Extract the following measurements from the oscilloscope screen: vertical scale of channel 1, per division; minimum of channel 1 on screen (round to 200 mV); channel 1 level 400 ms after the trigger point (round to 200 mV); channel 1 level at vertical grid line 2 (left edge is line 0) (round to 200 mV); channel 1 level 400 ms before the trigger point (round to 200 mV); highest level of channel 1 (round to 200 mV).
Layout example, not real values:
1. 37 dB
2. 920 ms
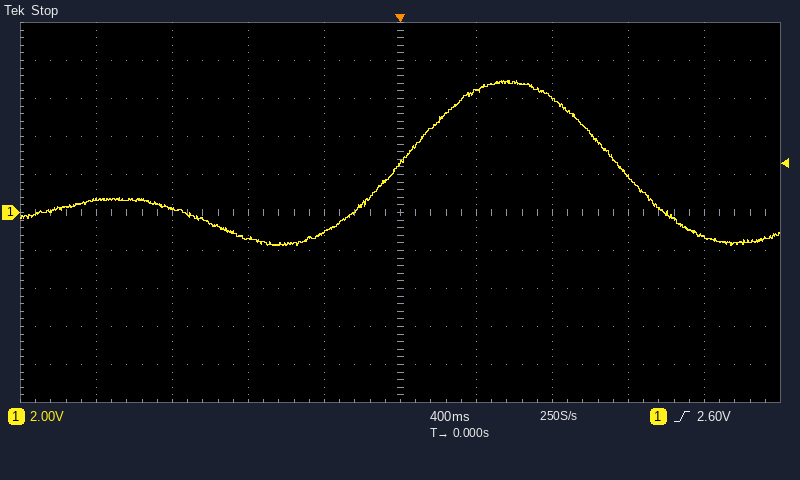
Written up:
1. 2 V
2. -1.8 V
3. 6.4 V
4. 200 mV
5. -1.0 V
6. 7.0 V
